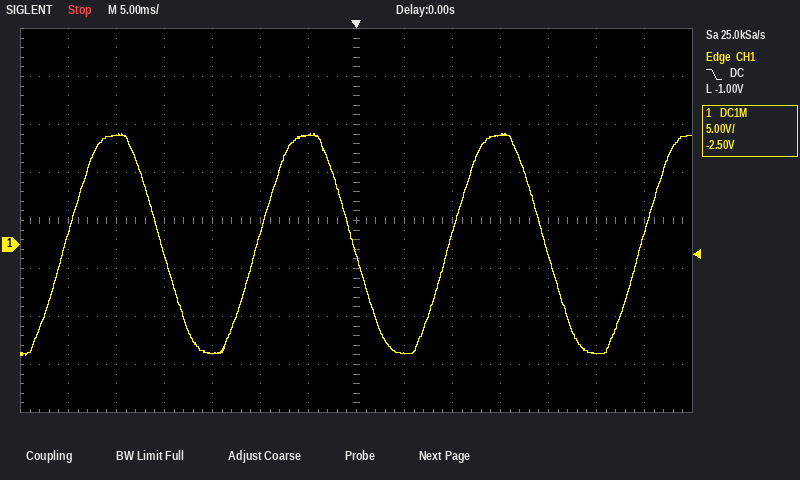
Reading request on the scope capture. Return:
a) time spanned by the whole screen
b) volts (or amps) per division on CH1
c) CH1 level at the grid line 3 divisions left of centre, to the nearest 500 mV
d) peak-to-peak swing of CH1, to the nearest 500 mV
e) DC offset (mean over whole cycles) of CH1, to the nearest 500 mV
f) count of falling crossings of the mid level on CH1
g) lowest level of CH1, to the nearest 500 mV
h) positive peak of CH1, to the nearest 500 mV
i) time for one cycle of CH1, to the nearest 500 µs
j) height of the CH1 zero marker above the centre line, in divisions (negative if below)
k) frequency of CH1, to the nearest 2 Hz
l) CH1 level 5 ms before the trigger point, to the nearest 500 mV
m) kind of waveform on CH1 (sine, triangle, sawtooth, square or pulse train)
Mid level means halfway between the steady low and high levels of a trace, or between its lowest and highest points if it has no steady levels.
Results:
70 ms
5 V
-11.5 V
23.0 V
0.0 V
3
-11.5 V
11.5 V
20.0 ms
-0.5 div
50 Hz
11.5 V
sine
